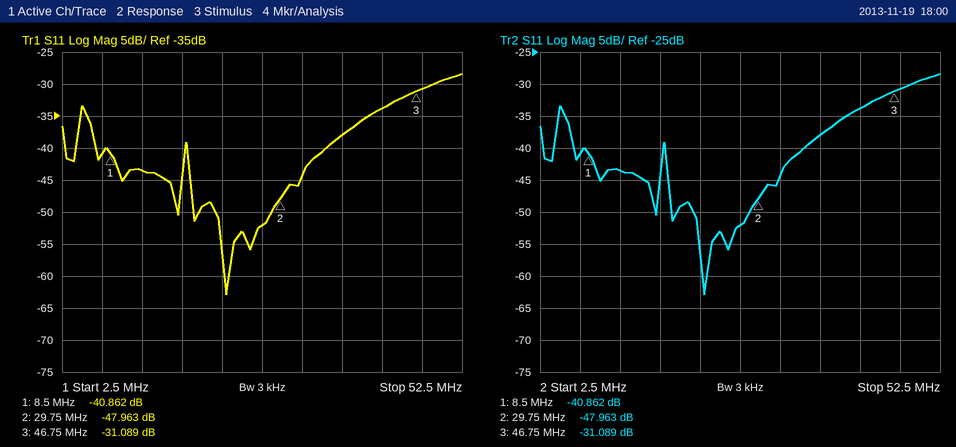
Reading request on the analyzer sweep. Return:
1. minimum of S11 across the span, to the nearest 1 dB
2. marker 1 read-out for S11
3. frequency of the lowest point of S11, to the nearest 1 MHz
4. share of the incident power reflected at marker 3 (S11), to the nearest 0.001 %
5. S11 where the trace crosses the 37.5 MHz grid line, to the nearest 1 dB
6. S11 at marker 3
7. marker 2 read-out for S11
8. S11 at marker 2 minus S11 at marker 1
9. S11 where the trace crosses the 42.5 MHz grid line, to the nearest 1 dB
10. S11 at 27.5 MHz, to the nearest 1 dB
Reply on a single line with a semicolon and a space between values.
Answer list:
-63 dB; -40.862 dB; 23 MHz; 0.078 %; -38 dB; -31.089 dB; -47.963 dB; -7.101 dB; -34 dB; -52 dB
